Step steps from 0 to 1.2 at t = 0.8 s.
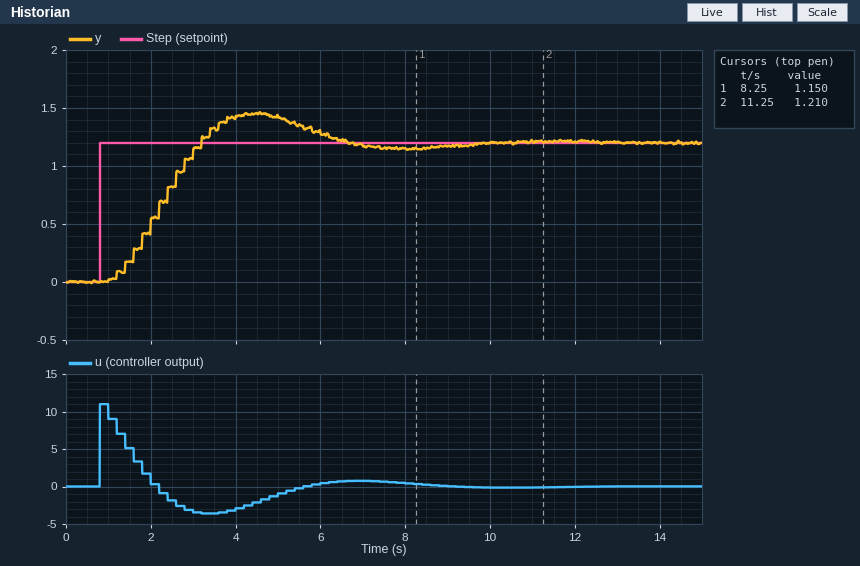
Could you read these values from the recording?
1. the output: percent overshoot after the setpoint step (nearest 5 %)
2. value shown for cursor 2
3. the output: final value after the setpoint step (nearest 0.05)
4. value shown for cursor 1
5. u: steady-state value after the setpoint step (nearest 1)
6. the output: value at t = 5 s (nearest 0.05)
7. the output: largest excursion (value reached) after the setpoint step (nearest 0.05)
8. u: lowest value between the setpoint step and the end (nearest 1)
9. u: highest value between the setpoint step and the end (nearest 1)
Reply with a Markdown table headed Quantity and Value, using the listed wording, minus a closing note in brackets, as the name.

| Quantity | Value |
|---|---|
| the output: percent overshoot after the setpoint step | 20 % |
| value shown for cursor 2 | 1.210 |
| the output: final value after the setpoint step | 1.20 |
| value shown for cursor 1 | 1.150 |
| u: steady-state value after the setpoint step | 0 |
| the output: value at t = 5 s | 1.40 |
| the output: largest excursion (value reached) after the setpoint step | 1.45 |
| u: lowest value between the setpoint step and the end | -4 |
| u: highest value between the setpoint step and the end | 11 |
